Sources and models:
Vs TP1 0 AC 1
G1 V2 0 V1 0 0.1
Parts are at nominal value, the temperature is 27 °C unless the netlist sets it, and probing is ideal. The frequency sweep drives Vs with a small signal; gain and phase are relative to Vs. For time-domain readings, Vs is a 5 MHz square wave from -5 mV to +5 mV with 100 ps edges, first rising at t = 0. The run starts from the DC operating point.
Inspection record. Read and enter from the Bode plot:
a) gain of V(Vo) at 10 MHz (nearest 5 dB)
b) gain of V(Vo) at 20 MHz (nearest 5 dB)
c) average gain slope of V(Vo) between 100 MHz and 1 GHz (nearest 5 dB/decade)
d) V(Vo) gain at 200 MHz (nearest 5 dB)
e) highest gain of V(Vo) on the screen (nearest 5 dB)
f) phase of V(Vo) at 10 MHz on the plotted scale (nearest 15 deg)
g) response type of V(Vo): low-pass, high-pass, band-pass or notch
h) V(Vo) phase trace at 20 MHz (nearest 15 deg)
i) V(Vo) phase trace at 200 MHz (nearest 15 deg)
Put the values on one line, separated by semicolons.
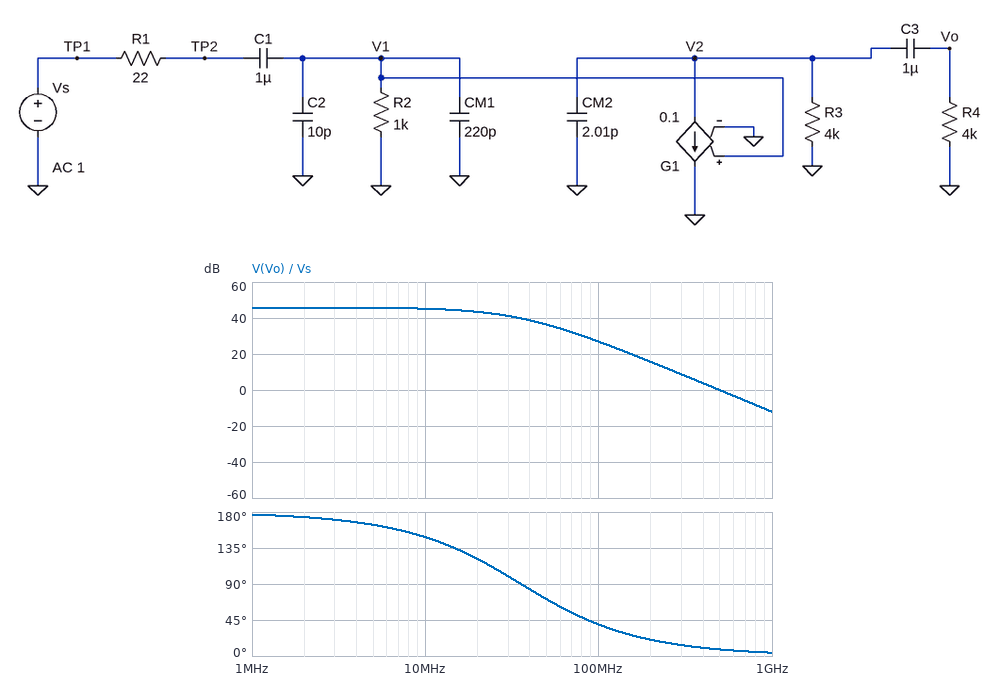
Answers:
45 dB; 45 dB; -40 dB/decade; 15 dB; 45 dB; 150 deg; low-pass; 120 deg; 15 deg
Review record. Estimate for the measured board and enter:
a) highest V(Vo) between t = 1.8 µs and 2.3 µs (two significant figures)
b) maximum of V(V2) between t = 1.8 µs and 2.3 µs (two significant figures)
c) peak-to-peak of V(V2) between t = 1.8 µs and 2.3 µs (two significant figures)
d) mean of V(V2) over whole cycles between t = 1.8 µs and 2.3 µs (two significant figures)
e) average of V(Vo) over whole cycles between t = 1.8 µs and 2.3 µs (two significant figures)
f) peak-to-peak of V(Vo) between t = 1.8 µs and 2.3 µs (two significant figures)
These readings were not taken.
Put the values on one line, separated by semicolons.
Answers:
2.4 mV; 1.8 mV; 2.0 V; -980 mV; -980 mV; 2.0 V
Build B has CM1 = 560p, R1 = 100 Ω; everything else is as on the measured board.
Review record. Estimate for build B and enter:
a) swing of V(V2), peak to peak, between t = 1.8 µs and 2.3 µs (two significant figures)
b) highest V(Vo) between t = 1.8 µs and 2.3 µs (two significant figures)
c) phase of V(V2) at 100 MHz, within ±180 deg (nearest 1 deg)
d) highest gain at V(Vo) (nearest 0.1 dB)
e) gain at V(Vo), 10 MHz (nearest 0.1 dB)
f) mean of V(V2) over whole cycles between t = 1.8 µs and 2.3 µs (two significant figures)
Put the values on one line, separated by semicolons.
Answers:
1.3 V; -250 mV; 23 deg; 45.2 dB; 34.3 dB; -910 mV
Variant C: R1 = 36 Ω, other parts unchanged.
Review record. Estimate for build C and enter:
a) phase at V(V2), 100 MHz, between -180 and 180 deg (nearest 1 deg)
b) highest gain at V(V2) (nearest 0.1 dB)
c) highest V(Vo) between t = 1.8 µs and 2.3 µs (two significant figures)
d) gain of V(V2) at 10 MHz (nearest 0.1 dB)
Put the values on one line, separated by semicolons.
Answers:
33 deg; 45.7 dB; 2.3 mV; 44.5 dB
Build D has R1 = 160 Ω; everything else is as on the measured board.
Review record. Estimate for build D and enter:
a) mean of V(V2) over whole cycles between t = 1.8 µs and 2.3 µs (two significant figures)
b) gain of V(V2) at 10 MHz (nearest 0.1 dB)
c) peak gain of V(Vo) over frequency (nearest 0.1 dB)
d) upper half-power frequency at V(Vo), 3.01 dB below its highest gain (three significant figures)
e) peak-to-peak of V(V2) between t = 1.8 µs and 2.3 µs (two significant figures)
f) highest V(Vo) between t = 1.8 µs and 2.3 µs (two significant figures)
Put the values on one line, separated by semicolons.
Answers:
-860 mV; 37.5 dB; 44.7 dB; 4.94 MHz; 1.6 V; -79 mV
